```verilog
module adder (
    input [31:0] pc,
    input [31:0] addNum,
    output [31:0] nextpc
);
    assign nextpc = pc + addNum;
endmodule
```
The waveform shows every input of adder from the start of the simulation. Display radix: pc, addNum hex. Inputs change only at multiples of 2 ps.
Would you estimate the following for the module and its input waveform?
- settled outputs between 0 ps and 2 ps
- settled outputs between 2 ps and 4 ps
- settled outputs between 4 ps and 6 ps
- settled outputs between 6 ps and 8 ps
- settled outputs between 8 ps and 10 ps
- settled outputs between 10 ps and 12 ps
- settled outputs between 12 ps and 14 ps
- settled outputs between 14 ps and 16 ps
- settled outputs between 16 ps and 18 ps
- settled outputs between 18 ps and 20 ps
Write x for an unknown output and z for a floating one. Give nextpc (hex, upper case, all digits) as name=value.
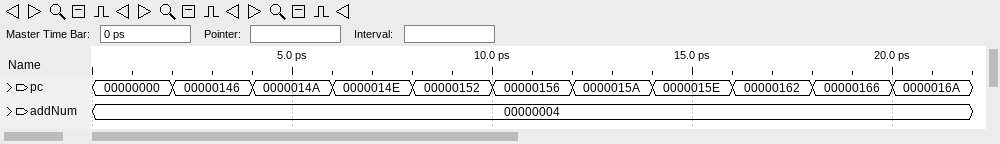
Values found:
nextpc=00000004
nextpc=0000014A
nextpc=0000014E
nextpc=00000152
nextpc=00000156
nextpc=0000015A
nextpc=0000015E
nextpc=00000162
nextpc=00000166
nextpc=0000016A
